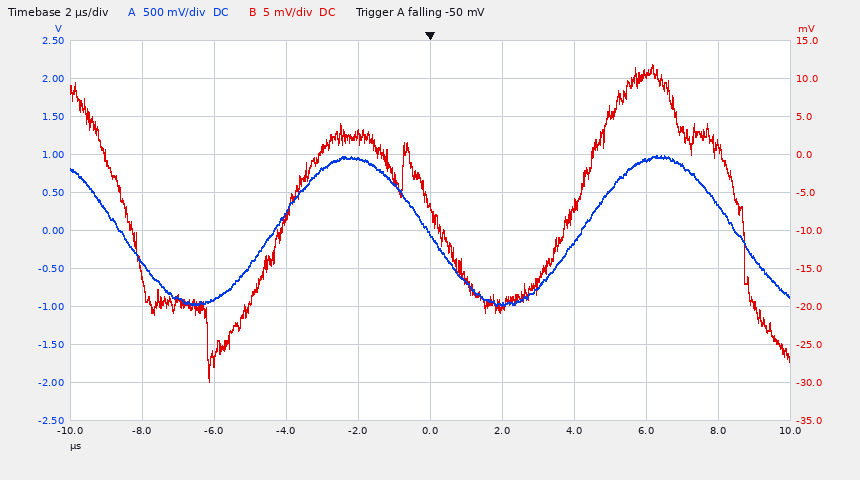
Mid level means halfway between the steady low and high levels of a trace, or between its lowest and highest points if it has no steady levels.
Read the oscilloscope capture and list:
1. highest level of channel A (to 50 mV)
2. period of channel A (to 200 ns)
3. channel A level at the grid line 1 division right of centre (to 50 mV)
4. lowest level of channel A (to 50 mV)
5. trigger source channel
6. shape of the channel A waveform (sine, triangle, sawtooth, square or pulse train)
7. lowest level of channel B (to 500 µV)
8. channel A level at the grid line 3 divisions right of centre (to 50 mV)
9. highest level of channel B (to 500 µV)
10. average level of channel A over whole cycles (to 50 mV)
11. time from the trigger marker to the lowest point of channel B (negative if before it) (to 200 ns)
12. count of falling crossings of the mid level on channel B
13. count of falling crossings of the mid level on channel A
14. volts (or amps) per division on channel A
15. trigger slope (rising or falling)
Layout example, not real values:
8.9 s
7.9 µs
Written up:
1.00 V
8.6 µs
-950 mV
-1.00 V
channel A
sine
-30.0 mV
950 mV
12.0 mV
0 mV
-6.2 µs
3
3
500 mV
falling
